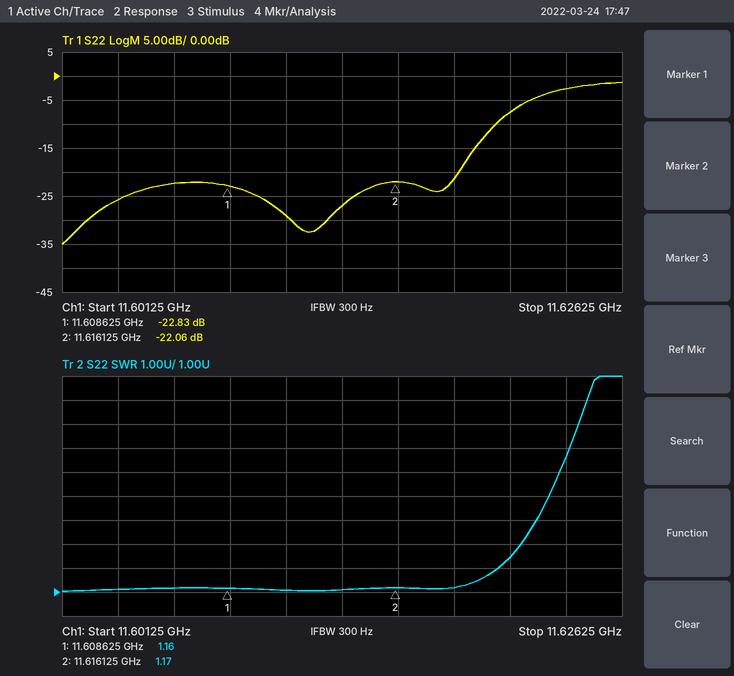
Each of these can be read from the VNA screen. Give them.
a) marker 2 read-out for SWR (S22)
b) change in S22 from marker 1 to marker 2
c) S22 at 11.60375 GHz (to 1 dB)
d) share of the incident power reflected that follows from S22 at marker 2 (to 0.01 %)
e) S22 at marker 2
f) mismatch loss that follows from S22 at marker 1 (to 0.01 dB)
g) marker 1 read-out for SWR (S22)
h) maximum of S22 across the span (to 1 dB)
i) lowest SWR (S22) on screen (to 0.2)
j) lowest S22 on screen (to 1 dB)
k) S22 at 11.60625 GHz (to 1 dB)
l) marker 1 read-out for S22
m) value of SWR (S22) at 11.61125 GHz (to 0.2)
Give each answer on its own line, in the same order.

1.17
0.77 dB
-26 dB
0.62 %
-22.06 dB
0.02 dB
1.16
-1 dB
1.0
-35 dB
-22 dB
-22.83 dB
1.0
